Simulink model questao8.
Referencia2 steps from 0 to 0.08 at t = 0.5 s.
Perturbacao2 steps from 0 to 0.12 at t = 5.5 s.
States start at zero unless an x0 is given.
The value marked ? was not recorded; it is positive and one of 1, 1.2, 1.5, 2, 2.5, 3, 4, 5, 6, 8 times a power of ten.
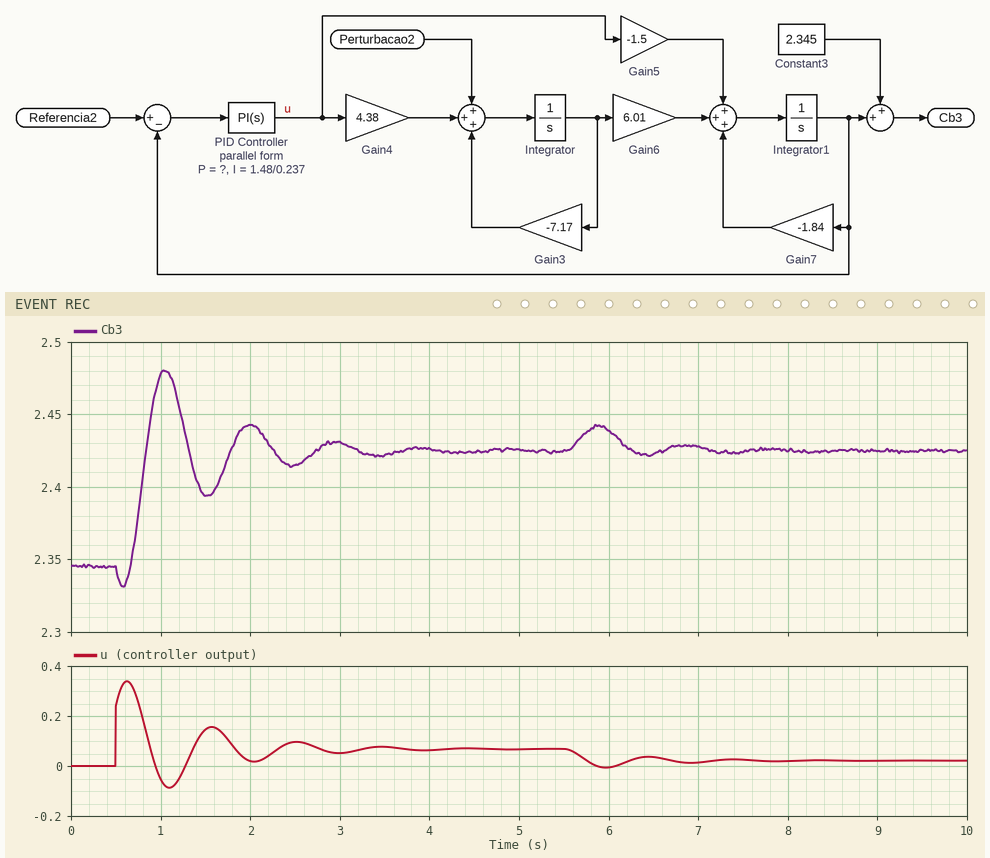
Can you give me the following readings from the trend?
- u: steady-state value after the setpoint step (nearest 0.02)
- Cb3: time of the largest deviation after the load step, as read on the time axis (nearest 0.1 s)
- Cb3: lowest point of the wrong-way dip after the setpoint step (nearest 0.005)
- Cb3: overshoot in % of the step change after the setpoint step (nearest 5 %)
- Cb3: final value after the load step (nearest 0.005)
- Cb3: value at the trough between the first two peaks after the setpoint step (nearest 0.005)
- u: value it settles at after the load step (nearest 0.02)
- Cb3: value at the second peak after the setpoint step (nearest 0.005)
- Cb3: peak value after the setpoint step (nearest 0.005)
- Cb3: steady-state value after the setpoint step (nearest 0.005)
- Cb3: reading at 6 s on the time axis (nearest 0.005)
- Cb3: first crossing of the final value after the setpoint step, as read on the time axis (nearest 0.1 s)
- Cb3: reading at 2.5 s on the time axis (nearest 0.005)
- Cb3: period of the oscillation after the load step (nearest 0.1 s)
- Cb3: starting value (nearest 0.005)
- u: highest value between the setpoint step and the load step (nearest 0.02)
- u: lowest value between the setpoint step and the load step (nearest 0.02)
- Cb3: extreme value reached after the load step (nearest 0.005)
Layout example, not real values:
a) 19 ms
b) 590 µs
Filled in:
a) 0.06
b) 5.9 s
c) 2.330
d) 70 %
e) 2.425
f) 2.395
g) 0.02
h) 2.445
i) 2.480
j) 2.425
k) 2.440
l) 0.8 s
m) 2.415
n) 1.0 s
o) 2.345
p) 0.34
q) -0.08
r) 2.440
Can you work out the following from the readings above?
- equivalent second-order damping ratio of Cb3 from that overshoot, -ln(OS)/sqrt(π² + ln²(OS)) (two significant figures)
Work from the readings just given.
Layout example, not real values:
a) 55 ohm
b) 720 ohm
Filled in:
a) 0.11
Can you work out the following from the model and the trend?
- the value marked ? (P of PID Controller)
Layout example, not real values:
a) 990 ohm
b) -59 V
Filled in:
a) 3
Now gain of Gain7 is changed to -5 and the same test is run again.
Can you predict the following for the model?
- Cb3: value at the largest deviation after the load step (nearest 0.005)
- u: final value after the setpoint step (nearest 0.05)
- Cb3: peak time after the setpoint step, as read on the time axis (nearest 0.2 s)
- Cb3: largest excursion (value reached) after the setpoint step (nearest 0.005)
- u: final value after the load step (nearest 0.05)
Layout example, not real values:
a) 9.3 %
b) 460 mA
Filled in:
a) 2.435
b) 0.20
c) 1.0 s
d) 2.430
e) 0.15
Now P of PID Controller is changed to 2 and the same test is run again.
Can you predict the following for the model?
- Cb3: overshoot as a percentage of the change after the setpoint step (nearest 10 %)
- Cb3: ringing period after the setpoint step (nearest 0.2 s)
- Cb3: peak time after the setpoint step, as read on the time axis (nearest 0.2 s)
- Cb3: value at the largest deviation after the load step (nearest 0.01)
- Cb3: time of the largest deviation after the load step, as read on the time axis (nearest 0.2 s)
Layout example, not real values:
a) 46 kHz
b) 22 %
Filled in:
a) 60 %
b) 1.2 s
c) 1.2 s
d) 2.44
e) 6.0 s
